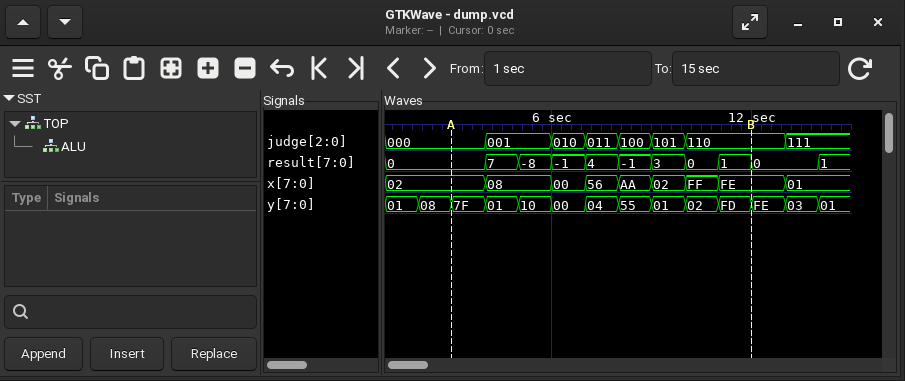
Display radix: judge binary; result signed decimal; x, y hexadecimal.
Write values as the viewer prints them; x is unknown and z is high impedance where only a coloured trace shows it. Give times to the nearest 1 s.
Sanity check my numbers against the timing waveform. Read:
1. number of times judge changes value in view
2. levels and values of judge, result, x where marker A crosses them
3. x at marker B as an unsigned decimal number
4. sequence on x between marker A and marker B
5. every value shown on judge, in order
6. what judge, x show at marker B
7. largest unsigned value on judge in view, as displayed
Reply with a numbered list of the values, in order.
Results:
1. 7
2. judge=000, result=0, x=02
3. 254
4. 02, 08, 00, 56, AA, 02, FF, FE
5. 000, 001, 010, 011, 100, 101, 110, 111
6. judge=110, x=FE
7. 111
